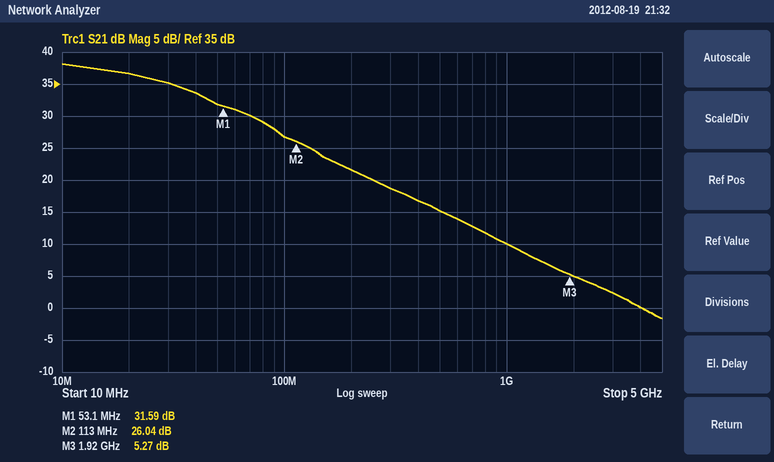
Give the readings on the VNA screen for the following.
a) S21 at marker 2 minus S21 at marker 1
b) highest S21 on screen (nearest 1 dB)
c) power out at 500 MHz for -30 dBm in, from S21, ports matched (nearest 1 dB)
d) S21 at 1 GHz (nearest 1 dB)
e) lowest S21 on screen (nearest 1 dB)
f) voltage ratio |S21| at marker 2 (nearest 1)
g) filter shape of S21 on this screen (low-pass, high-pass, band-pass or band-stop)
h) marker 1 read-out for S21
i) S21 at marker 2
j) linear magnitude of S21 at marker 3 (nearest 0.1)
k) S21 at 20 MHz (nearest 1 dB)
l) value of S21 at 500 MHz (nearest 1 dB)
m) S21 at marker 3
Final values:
-5.55 dB
38 dB
-15 dBm
10 dB
-2 dB
20
low-pass
31.59 dB
26.04 dB
1.8
37 dB
15 dB
5.27 dB
